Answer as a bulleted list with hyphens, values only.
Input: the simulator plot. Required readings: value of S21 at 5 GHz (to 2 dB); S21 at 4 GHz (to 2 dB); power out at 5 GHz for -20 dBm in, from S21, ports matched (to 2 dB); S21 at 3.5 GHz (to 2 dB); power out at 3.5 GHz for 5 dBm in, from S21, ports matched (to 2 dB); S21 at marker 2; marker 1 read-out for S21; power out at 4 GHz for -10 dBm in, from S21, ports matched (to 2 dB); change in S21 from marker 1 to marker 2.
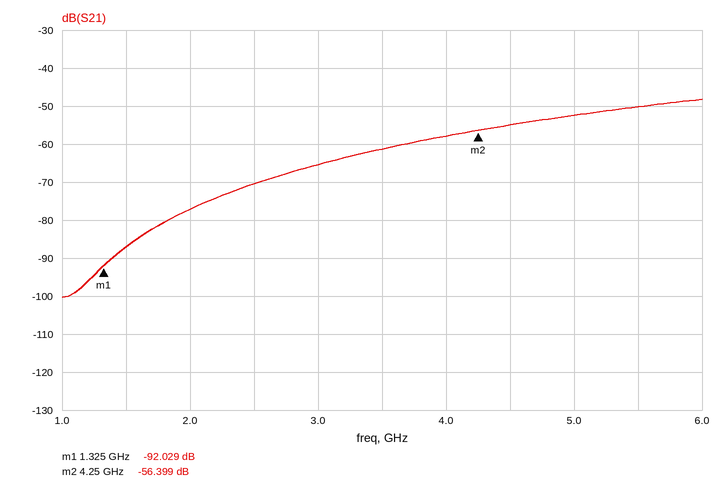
- -52 dB
- -58 dB
- -72 dBm
- -62 dB
- -56 dBm
- -56.399 dB
- -92.029 dB
- -68 dBm
- 35.630 dB
